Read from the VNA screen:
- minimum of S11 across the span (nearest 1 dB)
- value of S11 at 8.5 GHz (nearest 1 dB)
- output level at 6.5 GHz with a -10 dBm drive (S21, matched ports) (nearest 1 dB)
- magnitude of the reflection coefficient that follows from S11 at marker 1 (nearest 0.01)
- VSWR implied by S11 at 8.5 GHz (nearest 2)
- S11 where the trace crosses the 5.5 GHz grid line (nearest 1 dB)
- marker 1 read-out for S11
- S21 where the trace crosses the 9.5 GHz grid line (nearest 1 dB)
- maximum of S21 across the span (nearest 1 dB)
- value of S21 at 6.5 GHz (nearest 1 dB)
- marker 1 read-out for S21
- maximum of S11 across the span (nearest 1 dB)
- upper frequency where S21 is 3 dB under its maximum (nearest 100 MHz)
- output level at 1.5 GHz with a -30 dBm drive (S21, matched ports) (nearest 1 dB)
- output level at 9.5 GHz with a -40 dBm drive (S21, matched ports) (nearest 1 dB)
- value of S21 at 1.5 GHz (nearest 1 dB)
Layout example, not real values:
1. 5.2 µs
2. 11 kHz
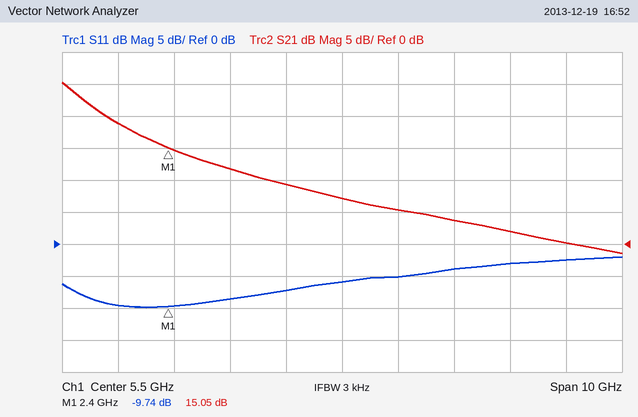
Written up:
1. -10 dB
2. -3 dB
3. -5 dBm
4. 0.33
5. 6
6. -6 dB
7. -9.74 dB
8. 0 dB
9. 25 dB
10. 5 dB
11. 15.05 dB
12. -2 dB
13. 900 MHz
14. -11 dBm
15. -40 dBm
16. 19 dB
